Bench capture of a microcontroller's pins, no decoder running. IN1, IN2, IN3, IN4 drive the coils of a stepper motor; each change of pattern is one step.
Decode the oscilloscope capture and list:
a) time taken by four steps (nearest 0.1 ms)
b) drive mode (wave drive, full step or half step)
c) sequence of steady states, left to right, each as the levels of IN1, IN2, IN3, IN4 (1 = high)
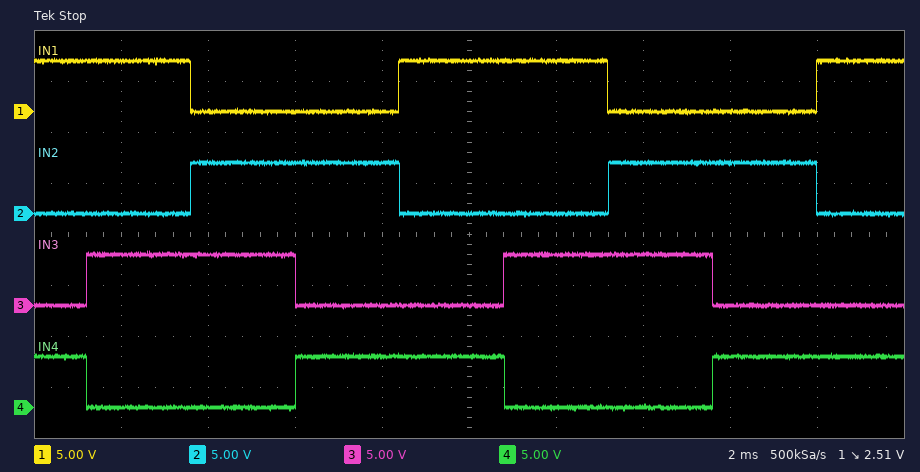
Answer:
9.6 ms
full step
1001 1010 0110 0101 1001 1010 0110 0101 1001
